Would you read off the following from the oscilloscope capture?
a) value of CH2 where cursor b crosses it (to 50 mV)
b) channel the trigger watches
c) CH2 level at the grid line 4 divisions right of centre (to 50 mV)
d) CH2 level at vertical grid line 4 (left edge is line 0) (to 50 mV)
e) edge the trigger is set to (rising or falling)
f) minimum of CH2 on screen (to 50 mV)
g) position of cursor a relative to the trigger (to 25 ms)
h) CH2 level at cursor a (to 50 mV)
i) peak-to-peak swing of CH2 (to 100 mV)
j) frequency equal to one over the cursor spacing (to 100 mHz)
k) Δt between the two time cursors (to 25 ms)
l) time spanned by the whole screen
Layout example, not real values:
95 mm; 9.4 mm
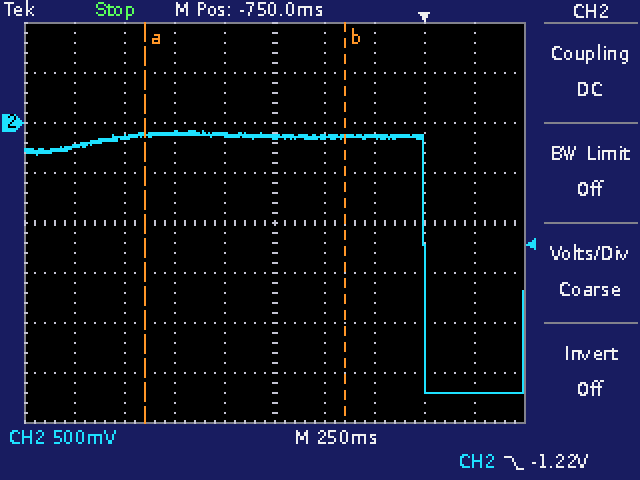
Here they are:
-150 mV; CH2; -2.70 V; -100 mV; falling; -2.70 V; -1.400 s; -100 mV; 2.60 V; 1.0 Hz; 1.000 s; 2.5 s
